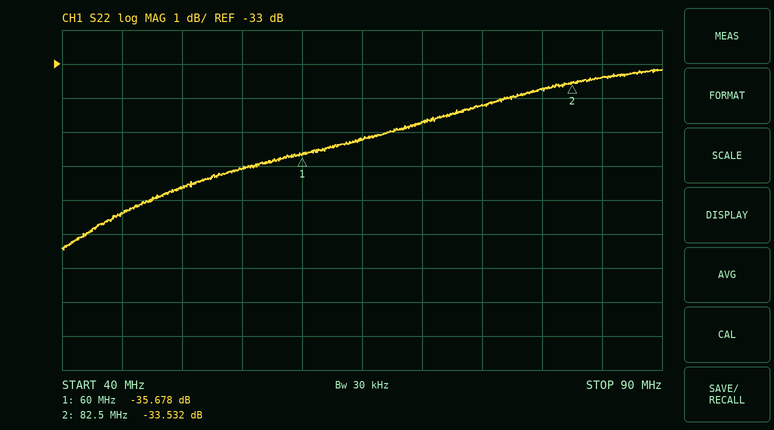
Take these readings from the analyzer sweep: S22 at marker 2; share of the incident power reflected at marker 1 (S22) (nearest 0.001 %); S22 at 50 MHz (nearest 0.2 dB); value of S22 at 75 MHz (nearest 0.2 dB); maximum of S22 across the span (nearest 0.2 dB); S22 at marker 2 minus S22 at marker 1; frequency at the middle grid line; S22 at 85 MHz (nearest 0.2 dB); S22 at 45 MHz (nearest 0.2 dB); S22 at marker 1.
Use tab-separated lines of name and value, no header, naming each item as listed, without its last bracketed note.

S22 at marker 2	-33.532 dB
share of the incident power reflected at marker 1 (S22)	0.027 %
S22 at 50 MHz	-36.6 dB
value of S22 at 75 MHz	-34.2 dB
maximum of S22 across the span	-33.2 dB
S22 at marker 2 minus S22 at marker 1	2.146 dB
frequency at the middle grid line	65 MHz
S22 at 85 MHz	-33.4 dB
S22 at 45 MHz	-37.4 dB
S22 at marker 1	-35.678 dB
